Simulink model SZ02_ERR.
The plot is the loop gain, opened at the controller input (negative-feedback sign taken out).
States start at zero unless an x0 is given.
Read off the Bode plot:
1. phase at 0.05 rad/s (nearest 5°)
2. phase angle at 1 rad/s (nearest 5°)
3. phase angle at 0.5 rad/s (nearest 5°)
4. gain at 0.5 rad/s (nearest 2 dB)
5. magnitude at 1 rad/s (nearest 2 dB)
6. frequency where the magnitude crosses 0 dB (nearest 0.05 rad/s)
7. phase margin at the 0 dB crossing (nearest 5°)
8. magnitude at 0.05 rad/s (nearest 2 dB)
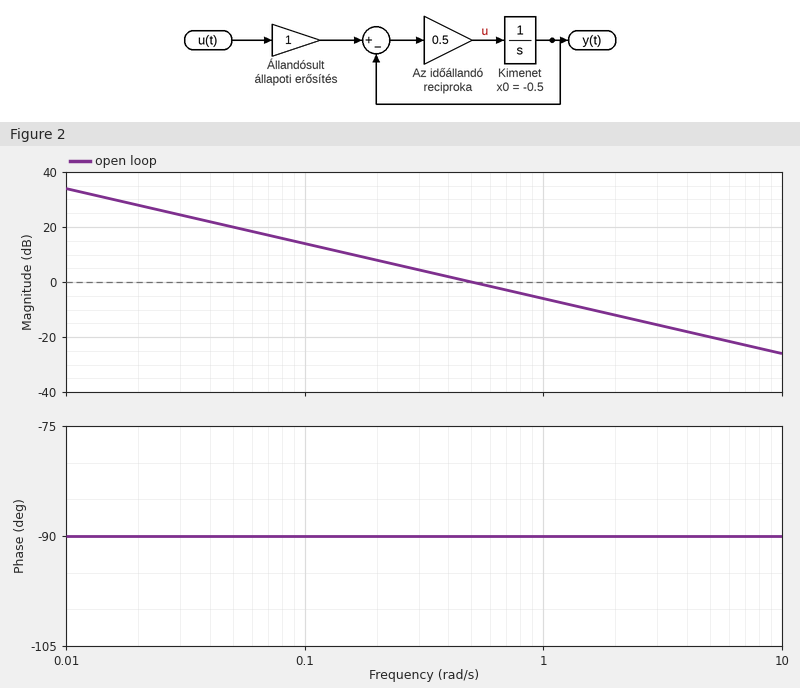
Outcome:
-90°
-90°
-90°
0 dB
-6 dB
0.50 rad/s
90°
20 dB
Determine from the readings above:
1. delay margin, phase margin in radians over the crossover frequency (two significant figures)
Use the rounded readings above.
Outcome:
3.1 s
